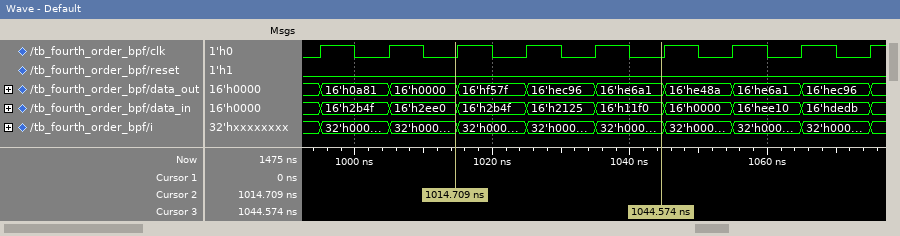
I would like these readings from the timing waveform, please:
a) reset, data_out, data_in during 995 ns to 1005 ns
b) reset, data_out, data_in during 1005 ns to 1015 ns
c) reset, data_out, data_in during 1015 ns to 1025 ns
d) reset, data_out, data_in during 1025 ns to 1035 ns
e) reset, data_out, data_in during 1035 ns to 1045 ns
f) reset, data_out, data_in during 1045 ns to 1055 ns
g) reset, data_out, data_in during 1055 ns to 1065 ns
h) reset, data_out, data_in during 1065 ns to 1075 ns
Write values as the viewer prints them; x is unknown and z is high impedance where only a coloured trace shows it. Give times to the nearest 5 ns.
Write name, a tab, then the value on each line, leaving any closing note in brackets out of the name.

reset, data_out, data_in during 995 ns to 1005 ns	reset=0, data_out=16'h0a81, data_in=16'h2b4f
reset, data_out, data_in during 1005 ns to 1015 ns	reset=0, data_out=16'h0000, data_in=16'h2ee0
reset, data_out, data_in during 1015 ns to 1025 ns	reset=0, data_out=16'hf57f, data_in=16'h2b4f
reset, data_out, data_in during 1025 ns to 1035 ns	reset=0, data_out=16'hec96, data_in=16'h2125
reset, data_out, data_in during 1035 ns to 1045 ns	reset=0, data_out=16'he6a1, data_in=16'h11f0
reset, data_out, data_in during 1045 ns to 1055 ns	reset=0, data_out=16'he48a, data_in=16'h0000
reset, data_out, data_in during 1055 ns to 1065 ns	reset=0, data_out=16'he6a1, data_in=16'hee10
reset, data_out, data_in during 1065 ns to 1075 ns	reset=0, data_out=16'hec96, data_in=16'hdedb
